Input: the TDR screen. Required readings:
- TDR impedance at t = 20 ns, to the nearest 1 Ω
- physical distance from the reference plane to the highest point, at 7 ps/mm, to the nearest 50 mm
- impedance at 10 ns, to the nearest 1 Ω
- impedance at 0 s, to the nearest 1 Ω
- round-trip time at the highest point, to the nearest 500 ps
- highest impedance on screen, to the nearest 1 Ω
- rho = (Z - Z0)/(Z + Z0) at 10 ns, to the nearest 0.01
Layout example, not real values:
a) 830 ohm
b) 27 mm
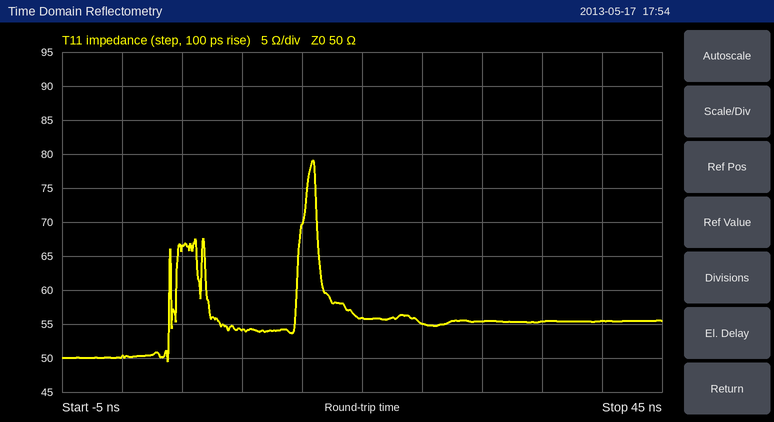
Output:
a) 56 Ω
b) 1.15 m
c) 54 Ω
d) 50 Ω
e) 16.0 ns
f) 79 Ω
g) +0.04
